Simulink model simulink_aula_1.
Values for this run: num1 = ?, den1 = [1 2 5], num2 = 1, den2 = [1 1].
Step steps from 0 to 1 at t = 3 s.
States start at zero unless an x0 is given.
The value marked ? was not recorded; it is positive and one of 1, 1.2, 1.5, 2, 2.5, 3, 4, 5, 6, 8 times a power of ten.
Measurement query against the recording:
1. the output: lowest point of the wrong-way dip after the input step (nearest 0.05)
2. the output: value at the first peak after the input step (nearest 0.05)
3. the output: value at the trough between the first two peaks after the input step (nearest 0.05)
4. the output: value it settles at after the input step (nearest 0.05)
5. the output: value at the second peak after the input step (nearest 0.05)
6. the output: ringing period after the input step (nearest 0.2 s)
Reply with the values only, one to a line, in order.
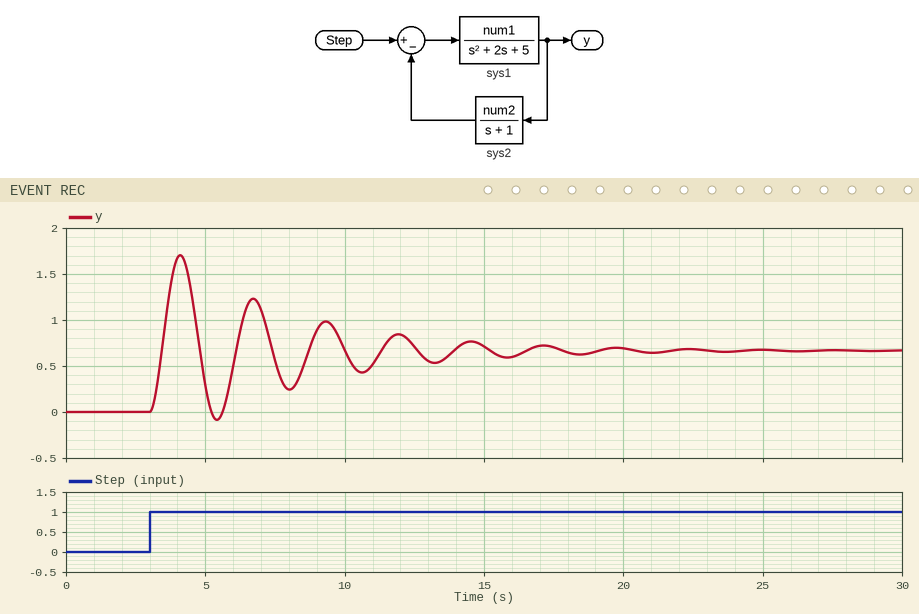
-0.10
1.70
-0.10
0.65
1.25
2.6 s
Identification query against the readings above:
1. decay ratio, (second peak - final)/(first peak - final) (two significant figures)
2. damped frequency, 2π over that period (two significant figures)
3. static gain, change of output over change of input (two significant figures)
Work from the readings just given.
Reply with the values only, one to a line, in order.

0.57
2.4 rad/s
0.65
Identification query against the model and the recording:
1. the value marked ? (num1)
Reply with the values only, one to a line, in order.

10
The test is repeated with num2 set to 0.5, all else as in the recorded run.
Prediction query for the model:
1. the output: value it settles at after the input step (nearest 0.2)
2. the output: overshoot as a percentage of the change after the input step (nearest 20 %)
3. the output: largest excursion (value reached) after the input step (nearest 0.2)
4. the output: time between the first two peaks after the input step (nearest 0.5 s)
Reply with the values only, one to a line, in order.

1.0
100 %
2.0
3.0 s
